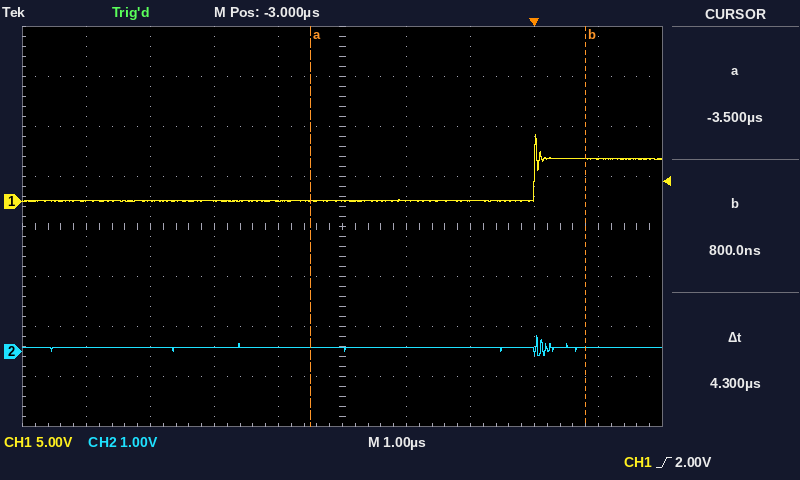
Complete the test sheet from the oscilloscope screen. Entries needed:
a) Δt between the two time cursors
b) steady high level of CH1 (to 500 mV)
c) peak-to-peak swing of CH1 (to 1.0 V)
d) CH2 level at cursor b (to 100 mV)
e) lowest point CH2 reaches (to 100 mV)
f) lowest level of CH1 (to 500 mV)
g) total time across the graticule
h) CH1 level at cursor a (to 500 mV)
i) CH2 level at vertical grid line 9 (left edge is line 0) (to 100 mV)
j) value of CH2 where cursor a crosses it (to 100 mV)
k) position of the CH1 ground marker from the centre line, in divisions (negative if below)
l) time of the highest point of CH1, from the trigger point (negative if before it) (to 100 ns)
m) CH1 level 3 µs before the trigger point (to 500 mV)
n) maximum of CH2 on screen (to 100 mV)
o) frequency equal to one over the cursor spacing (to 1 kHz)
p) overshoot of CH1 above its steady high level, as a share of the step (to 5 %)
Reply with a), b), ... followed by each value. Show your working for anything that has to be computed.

a) 4.3 µs
b) 4.5 V
c) 7.0 V
d) 100 mV
e) -100 mV
f) 0.0 V
g) 10 µs
h) 0.0 V
i) 100 mV
j) 100 mV
k) +0.5 div
l) 0.0 µs
m) 0.0 V
n) 300 mV
o) 1 / 4.3 µs ≈ 233 kHz
p) 55 %
